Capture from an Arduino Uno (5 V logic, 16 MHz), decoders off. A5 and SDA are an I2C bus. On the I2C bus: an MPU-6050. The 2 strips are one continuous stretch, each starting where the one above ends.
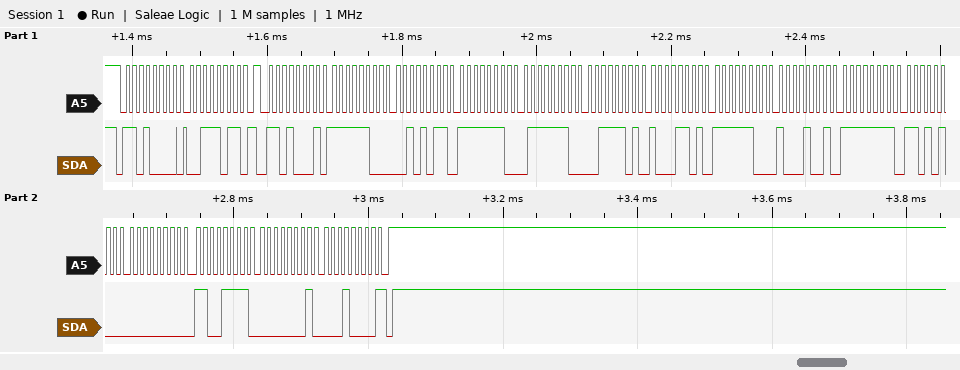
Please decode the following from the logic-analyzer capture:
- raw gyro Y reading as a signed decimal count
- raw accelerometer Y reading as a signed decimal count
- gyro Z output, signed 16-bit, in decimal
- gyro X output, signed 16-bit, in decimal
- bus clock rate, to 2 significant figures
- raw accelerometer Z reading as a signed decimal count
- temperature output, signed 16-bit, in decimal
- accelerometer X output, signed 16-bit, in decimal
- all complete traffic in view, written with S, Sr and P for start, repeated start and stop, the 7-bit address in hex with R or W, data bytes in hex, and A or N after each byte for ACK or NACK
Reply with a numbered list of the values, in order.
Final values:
1. 207
2. -386
3. 272
4. -44
5. 100 kHz
6. 15757
7. -887
8. -981
9. S 68W A 3B A Sr 68R A FC A 2B A FE A 7E A 3D A 8D A FC A 89 A FF A D4 A 00 A CF A 01 A 10 N P
